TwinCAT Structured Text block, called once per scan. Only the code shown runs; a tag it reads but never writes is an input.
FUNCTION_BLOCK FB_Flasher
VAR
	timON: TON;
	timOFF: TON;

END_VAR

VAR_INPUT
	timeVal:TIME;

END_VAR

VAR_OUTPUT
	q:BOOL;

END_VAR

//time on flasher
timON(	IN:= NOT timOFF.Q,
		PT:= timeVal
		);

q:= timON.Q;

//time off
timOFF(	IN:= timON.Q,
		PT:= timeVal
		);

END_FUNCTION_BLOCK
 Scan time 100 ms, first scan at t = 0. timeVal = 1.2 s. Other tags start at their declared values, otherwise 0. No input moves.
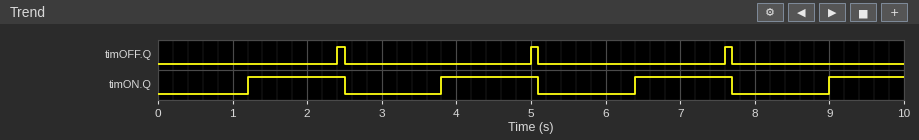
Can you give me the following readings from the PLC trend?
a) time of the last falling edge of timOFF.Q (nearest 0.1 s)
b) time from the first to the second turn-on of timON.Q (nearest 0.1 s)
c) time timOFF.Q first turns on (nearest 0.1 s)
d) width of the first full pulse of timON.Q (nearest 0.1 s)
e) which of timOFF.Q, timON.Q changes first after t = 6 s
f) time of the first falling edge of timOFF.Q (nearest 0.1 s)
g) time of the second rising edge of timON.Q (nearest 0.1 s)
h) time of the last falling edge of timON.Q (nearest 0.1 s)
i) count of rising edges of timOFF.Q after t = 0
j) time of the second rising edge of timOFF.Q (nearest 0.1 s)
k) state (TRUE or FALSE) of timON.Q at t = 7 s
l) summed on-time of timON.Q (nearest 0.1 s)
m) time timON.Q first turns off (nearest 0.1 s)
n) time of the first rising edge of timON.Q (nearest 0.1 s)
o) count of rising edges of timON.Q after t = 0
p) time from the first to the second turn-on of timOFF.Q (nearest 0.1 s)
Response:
7.7 s
2.6 s
2.4 s
1.3 s
timON.Q
2.5 s
3.8 s
7.7 s
3
5.0 s
TRUE
4.9 s
2.5 s
1.2 s
4
2.6 s
